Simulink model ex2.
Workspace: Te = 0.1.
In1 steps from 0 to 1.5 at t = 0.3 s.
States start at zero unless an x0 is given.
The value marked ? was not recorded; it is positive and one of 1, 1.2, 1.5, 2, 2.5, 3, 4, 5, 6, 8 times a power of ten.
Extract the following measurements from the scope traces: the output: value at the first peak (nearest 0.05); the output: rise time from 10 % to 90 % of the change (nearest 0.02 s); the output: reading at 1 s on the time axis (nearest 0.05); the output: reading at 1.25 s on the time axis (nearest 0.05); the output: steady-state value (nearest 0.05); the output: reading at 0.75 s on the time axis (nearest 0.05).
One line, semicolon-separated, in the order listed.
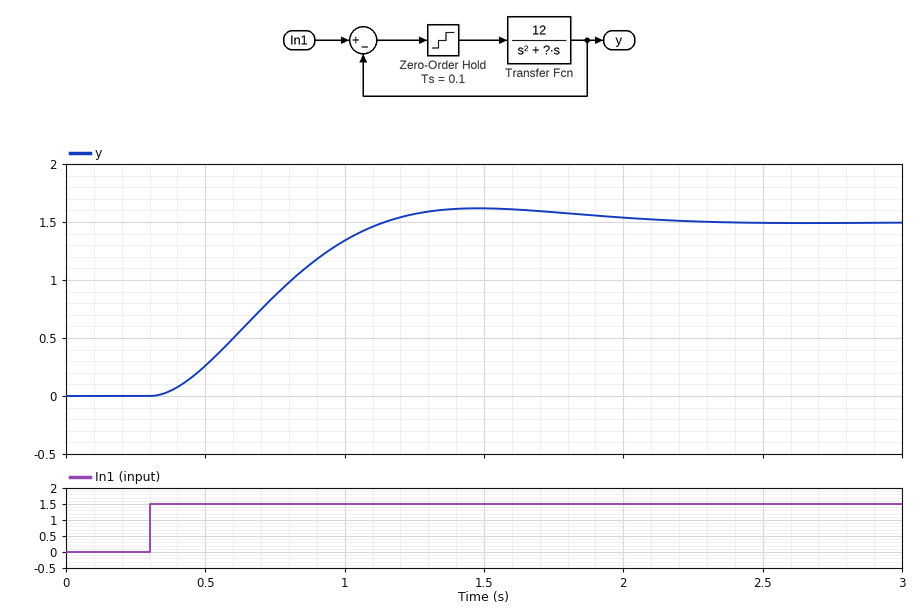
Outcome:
1.60; 0.56 s; 1.35; 1.55; 1.50; 0.85
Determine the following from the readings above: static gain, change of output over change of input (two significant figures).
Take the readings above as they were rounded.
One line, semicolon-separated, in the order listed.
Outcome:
1.0
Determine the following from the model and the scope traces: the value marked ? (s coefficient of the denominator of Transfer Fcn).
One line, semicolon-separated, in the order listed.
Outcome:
5
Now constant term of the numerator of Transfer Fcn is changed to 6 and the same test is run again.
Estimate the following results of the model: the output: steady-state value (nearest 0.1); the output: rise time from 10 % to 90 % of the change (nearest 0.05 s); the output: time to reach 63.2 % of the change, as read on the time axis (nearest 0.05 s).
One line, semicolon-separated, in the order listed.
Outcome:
1.5; 1.30 s; 1.15 s
